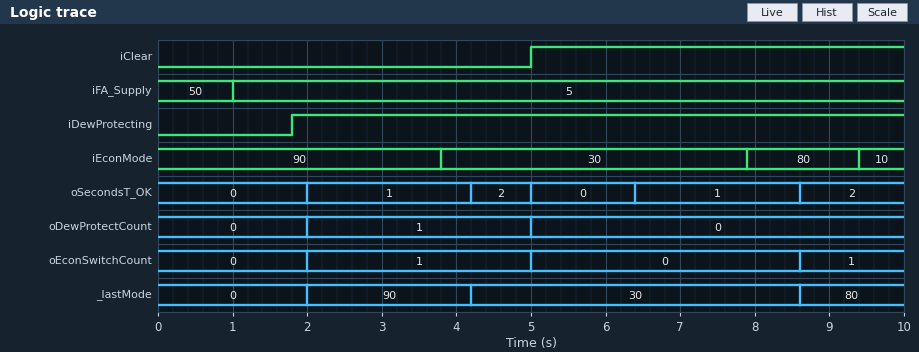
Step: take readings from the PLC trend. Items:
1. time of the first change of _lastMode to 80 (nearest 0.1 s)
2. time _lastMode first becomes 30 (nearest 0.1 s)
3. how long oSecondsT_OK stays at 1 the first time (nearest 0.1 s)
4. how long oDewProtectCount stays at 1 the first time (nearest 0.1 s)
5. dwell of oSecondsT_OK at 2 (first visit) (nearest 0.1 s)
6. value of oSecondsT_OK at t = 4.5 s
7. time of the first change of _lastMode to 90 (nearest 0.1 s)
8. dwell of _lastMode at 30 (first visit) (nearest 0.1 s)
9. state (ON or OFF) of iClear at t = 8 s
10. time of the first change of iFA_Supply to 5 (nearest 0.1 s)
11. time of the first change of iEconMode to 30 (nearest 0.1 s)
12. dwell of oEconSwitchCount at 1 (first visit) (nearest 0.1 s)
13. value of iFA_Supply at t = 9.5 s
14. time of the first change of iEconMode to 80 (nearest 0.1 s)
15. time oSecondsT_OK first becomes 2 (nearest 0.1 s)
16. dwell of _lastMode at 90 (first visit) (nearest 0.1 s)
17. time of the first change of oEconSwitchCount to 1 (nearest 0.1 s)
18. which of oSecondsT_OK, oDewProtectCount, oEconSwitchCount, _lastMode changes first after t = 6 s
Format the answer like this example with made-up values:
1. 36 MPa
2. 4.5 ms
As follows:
1. 8.6 s
2. 4.2 s
3. 2.2 s
4. 3.0 s
5. 0.8 s
6. 2
7. 2.0 s
8. 4.4 s
9. ON
10. 1.0 s
11. 3.8 s
12. 3.0 s
13. 5
14. 7.9 s
15. 4.2 s
16. 2.2 s
17. 2.0 s
18. oSecondsT_OK
